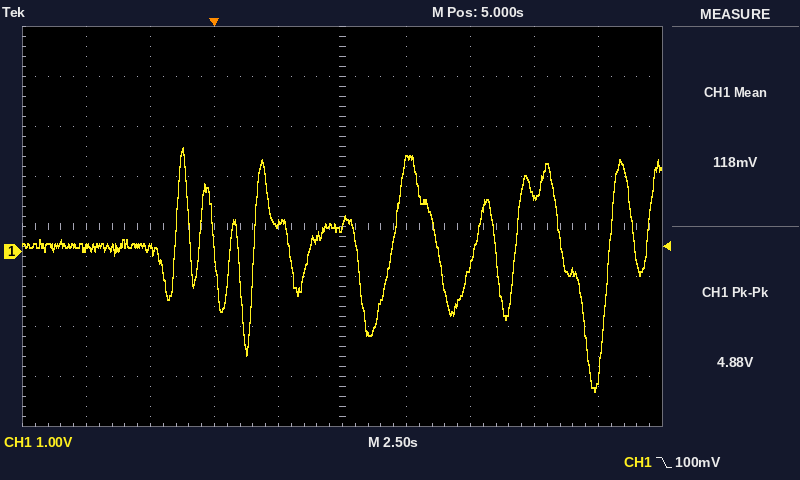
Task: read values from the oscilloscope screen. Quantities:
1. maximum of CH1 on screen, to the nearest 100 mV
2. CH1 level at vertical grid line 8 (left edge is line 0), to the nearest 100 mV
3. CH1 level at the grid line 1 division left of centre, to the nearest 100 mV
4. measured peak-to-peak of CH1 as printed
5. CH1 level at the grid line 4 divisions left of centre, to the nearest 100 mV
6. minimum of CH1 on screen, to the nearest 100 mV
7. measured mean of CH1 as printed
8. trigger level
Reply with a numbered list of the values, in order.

1. 2.1 V
2. 1.1 V
3. 600 mV
4. 4.88 V
5. 100 mV
6. -2.8 V
7. 118 mV
8. 100 mV
